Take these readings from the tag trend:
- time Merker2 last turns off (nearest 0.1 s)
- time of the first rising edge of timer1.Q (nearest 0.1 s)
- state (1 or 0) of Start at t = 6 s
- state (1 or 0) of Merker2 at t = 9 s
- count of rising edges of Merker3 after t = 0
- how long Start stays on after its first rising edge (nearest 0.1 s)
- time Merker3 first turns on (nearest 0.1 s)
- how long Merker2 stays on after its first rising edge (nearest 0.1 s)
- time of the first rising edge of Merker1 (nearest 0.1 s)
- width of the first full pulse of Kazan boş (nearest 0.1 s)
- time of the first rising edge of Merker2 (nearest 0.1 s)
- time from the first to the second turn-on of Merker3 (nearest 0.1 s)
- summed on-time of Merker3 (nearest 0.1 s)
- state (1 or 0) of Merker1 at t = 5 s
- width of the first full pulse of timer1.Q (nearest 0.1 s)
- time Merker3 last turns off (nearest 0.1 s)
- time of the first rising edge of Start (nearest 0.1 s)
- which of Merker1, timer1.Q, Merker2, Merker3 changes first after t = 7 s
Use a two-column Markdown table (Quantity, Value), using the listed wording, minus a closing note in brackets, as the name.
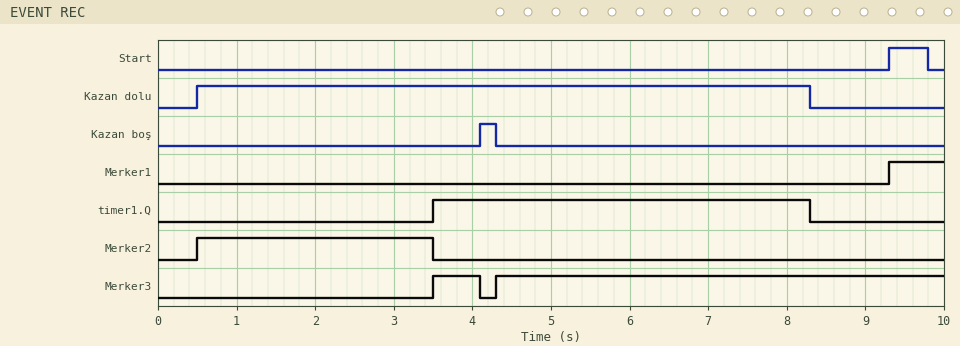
| Quantity | Value |
|---|---|
| time Merker2 last turns off | 3.5 s |
| time of the first rising edge of timer1.Q | 3.5 s |
| state (1 or 0) of Start at t = 6 s | 0 |
| state (1 or 0) of Merker2 at t = 9 s | 0 |
| count of rising edges of Merker3 after t = 0 | 2 |
| how long Start stays on after its first rising edge | 0.5 s |
| time Merker3 first turns on | 3.5 s |
| how long Merker2 stays on after its first rising edge | 3.0 s |
| time of the first rising edge of Merker1 | 9.3 s |
| width of the first full pulse of Kazan boş | 0.2 s |
| time of the first rising edge of Merker2 | 0.5 s |
| time from the first to the second turn-on of Merker3 | 0.8 s |
| summed on-time of Merker3 | 6.3 s |
| state (1 or 0) of Merker1 at t = 5 s | 0 |
| width of the first full pulse of timer1.Q | 4.8 s |
| time Merker3 last turns off | 4.1 s |
| time of the first rising edge of Start | 9.3 s |
| which of Merker1, timer1.Q, Merker2, Merker3 changes first after t = 7 s | timer1.Q |
